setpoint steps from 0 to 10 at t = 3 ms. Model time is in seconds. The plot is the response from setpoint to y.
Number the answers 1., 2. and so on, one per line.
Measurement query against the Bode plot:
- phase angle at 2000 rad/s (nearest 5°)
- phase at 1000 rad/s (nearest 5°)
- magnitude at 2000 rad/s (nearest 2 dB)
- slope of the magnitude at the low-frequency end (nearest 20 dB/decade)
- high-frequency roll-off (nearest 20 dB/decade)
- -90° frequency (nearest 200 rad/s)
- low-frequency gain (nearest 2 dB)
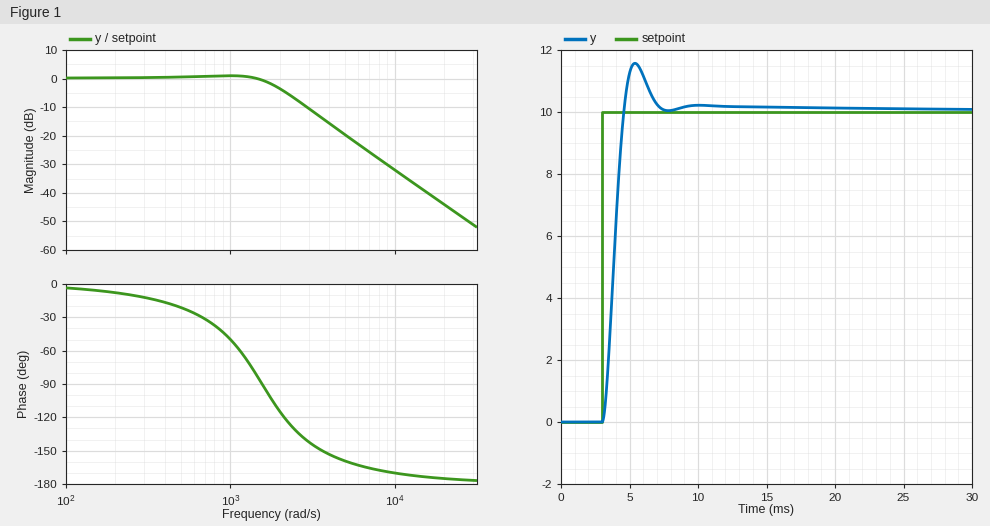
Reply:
1. -115°
2. -50°
3. -4 dB
4. 0 dB/decade
5. -40 dB/decade
6. 1600 rad/s
7. 0 dB
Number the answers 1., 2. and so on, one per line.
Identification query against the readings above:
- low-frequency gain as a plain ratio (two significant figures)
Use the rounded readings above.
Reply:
1. 1.0
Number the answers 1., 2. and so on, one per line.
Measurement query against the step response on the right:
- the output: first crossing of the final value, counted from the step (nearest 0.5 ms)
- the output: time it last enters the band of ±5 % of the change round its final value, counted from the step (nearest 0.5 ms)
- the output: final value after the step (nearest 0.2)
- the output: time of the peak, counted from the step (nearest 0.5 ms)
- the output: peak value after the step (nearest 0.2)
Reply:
1. 1.5 ms
2. 3.5 ms
3. 10.0
4. 2.5 ms
5. 11.6
